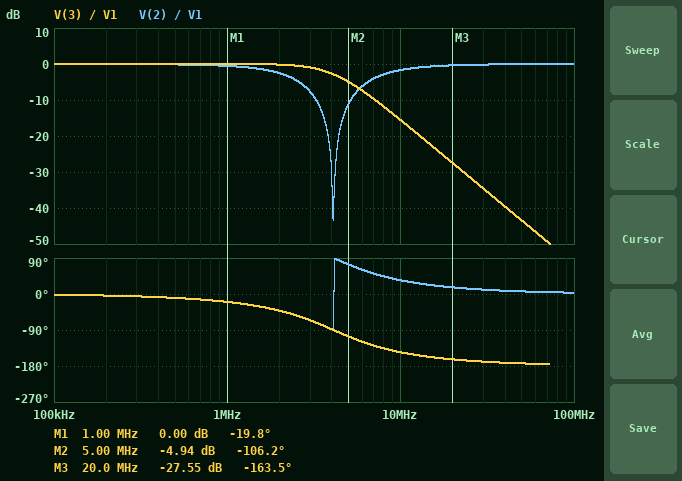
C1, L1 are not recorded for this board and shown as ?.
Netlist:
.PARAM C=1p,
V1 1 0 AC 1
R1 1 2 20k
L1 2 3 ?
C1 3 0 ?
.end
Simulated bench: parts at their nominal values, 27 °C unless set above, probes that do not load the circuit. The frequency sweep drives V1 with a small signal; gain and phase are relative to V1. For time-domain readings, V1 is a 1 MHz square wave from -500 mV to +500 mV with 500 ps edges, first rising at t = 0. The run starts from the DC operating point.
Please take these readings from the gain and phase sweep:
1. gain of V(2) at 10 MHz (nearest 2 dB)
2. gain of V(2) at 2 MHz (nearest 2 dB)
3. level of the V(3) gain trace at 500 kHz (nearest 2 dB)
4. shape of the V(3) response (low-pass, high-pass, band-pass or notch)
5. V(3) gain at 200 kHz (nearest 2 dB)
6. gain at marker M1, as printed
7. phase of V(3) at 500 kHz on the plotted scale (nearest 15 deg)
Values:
-2 dB
-2 dB
0 dB
low-pass
0 dB
0.00 dB
-15 deg
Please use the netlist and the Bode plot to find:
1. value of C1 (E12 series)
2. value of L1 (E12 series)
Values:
2.7 pF
560 µH
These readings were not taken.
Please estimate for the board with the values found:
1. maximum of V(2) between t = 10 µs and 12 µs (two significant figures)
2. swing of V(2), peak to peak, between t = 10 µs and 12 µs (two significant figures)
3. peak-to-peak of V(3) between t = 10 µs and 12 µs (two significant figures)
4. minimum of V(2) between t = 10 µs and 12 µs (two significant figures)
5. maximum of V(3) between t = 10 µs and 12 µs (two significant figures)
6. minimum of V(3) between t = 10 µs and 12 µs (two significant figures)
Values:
530 mV
1.1 V
1.1 V
-530 mV
550 mV
-550 mV
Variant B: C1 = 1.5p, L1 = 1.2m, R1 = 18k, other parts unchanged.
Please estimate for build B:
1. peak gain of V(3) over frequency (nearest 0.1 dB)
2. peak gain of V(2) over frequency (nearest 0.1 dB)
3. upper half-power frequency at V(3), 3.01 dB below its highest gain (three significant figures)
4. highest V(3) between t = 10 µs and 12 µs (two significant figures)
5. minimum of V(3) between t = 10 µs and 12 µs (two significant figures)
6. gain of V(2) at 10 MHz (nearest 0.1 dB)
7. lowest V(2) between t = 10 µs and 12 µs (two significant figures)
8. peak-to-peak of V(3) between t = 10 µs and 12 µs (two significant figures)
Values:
4.4 dB
0 dB
4.44 MHz
850 mV
-850 mV
-0.3 dB
-650 mV
1.7 V
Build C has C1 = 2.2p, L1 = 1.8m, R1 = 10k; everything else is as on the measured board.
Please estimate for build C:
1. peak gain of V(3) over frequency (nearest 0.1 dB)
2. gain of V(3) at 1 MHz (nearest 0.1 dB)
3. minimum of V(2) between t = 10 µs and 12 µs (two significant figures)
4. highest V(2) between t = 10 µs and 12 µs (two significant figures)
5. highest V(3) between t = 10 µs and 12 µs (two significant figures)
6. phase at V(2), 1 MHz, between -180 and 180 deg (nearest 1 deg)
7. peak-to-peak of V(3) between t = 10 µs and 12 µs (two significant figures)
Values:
9.3 dB
1.4 dB
-640 mV
640 mV
1.0 V
-9 deg
2.1 V
